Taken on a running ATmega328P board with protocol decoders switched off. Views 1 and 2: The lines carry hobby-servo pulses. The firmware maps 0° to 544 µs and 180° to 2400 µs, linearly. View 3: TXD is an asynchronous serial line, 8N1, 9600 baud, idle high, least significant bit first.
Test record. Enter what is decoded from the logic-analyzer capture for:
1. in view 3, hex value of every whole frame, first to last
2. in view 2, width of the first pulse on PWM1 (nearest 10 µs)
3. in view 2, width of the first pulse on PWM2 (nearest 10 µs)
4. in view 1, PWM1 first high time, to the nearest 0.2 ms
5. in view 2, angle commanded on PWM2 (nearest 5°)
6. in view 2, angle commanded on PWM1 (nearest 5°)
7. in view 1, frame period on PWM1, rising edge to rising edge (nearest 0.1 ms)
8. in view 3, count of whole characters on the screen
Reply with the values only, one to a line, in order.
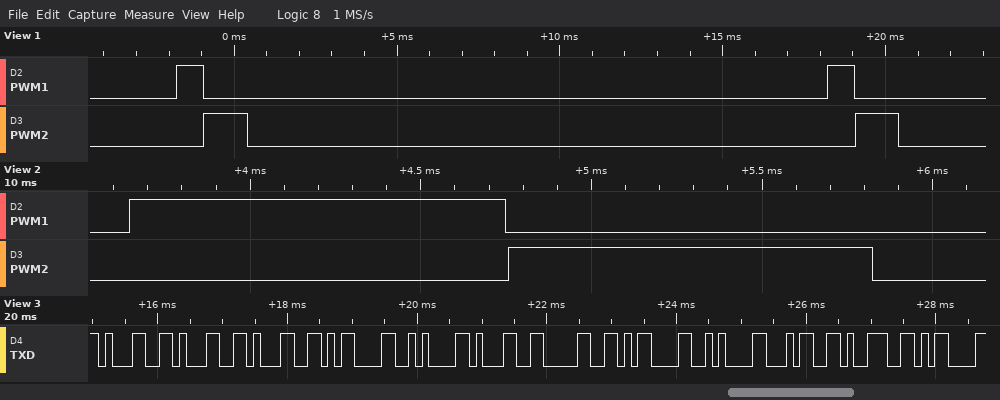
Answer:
0x31 0x31 0x31 0x0D 0x0A 0x31 0x30 0x0D 0x0A 0x34 0x39 0x0D
1100 µs
1070 µs
0.8 ms
50°
55°
20.0 ms
12
